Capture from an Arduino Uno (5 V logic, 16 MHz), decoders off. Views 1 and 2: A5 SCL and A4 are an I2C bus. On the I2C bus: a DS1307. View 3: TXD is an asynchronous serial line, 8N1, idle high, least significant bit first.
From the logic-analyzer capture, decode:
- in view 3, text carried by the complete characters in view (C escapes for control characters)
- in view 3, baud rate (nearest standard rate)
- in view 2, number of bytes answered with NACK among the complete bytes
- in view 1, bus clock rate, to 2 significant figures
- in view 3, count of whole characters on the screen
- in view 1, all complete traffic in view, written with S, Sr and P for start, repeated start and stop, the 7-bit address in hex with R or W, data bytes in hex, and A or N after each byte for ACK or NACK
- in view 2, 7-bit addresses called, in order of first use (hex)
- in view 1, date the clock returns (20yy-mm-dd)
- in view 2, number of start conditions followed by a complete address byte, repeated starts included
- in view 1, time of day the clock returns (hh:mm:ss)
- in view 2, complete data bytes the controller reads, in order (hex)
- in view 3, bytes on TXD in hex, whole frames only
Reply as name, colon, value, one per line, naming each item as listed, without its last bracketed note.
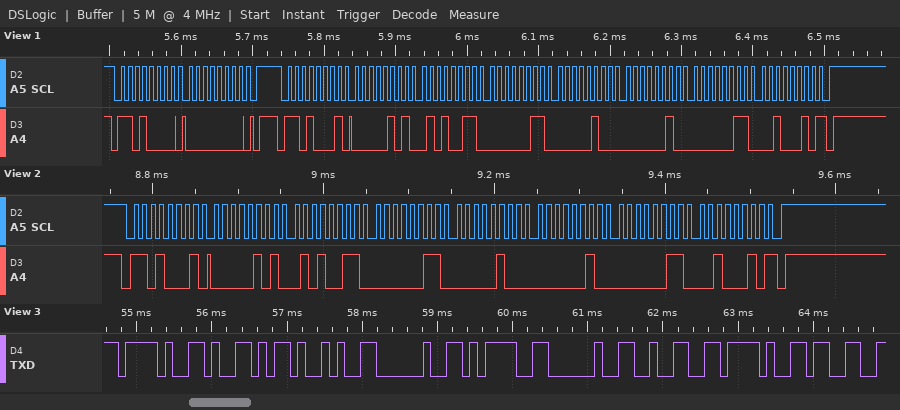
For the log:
in view 3, text carried by the complete characters in view: "/Y) = 2/3"
in view 3, baud rate: 9600 baud
in view 2, number of bytes answered with NACK among the complete bytes: 1
in view 1, bus clock rate, to 2 significant figures: 100 kHz
in view 3, count of whole characters on the screen: 9
in view 1, all complete traffic in view, written with S, Sr and P for start, repeated start and stop, the 7-bit address in hex with R or W, data bytes in hex, and A or N after each byte for ACK or NACK: S 68W A 00 A P S 68R A 05 A 53 A 03 A 04 A 02 A 03 A 22 N P
in view 2, 7-bit addresses called, in order of first use: 0x68
in view 1, date the clock returns: 2022-03-02
in view 2, number of start conditions followed by a complete address byte, repeated starts included: 1
in view 1, time of day the clock returns: 03:53:05
in view 2, complete data bytes the controller reads, in order: 05 53 03 04 02 03 22
in view 3, bytes on TXD in hex, whole frames only: 2F 59 29 20 3D 20 32 2F 33
